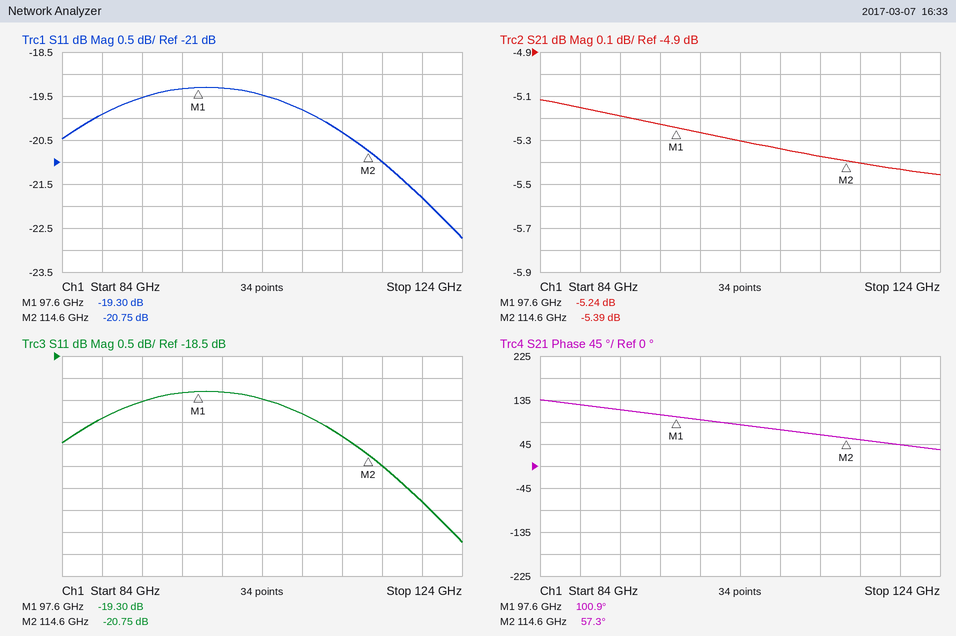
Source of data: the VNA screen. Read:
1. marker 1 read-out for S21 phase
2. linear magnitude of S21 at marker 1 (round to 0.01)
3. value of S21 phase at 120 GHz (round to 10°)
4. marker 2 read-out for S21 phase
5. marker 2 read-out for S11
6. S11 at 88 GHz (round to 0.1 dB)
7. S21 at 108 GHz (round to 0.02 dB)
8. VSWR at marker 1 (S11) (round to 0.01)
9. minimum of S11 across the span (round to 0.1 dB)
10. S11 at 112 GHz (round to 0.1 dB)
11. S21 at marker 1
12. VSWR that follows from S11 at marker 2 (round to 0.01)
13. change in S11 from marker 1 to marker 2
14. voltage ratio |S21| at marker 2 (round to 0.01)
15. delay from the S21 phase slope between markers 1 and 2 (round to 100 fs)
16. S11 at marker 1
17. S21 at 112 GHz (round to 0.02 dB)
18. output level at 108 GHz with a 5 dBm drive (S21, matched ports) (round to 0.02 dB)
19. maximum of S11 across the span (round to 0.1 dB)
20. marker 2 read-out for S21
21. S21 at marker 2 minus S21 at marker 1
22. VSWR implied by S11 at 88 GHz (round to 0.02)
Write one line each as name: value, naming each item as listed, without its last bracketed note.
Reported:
marker 1 read-out for S21 phase: 100.9°
linear magnitude of S21 at marker 1: 0.55
value of S21 phase at 120 GHz: 40°
marker 2 read-out for S21 phase: 57.3°
marker 2 read-out for S11: -20.75 dB
S11 at 88 GHz: -19.9 dB
S21 at 108 GHz: -5.34 dB
VSWR at marker 1 (S11): 1.24
minimum of S11 across the span: -22.7 dB
S11 at 112 GHz: -20.3 dB
S21 at marker 1: -5.24 dB
VSWR that follows from S11 at marker 2: 1.20
change in S11 from marker 1 to marker 2: -1.45 dB
voltage ratio |S21| at marker 2: 0.54
delay from the S21 phase slope between markers 1 and 2: 7.1 ps
S11 at marker 1: -19.30 dB
S21 at 112 GHz: -5.38 dB
output level at 108 GHz with a 5 dBm drive (S21, matched ports): -0.34 dBm
maximum of S11 across the span: -19.3 dB
marker 2 read-out for S21: -5.39 dB
S21 at marker 2 minus S21 at marker 1: -0.15 dB
VSWR implied by S11 at 88 GHz: 1.22
